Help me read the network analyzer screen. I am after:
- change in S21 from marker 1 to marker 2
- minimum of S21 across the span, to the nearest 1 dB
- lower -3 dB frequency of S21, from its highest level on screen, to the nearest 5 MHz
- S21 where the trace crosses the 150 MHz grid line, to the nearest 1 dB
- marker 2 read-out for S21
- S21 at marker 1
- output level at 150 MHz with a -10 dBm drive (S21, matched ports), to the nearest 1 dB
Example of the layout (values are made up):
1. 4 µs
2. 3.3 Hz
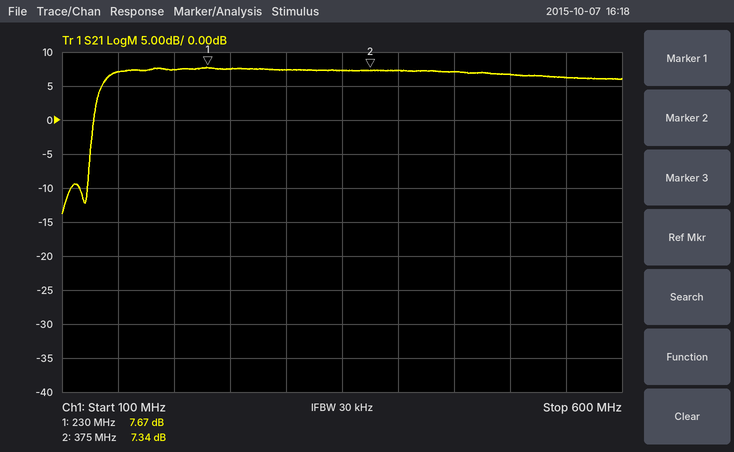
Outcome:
1. -0.33 dB
2. -14 dB
3. 135 MHz
4. 7 dB
5. 7.34 dB
6. 7.67 dB
7. -3 dBm
